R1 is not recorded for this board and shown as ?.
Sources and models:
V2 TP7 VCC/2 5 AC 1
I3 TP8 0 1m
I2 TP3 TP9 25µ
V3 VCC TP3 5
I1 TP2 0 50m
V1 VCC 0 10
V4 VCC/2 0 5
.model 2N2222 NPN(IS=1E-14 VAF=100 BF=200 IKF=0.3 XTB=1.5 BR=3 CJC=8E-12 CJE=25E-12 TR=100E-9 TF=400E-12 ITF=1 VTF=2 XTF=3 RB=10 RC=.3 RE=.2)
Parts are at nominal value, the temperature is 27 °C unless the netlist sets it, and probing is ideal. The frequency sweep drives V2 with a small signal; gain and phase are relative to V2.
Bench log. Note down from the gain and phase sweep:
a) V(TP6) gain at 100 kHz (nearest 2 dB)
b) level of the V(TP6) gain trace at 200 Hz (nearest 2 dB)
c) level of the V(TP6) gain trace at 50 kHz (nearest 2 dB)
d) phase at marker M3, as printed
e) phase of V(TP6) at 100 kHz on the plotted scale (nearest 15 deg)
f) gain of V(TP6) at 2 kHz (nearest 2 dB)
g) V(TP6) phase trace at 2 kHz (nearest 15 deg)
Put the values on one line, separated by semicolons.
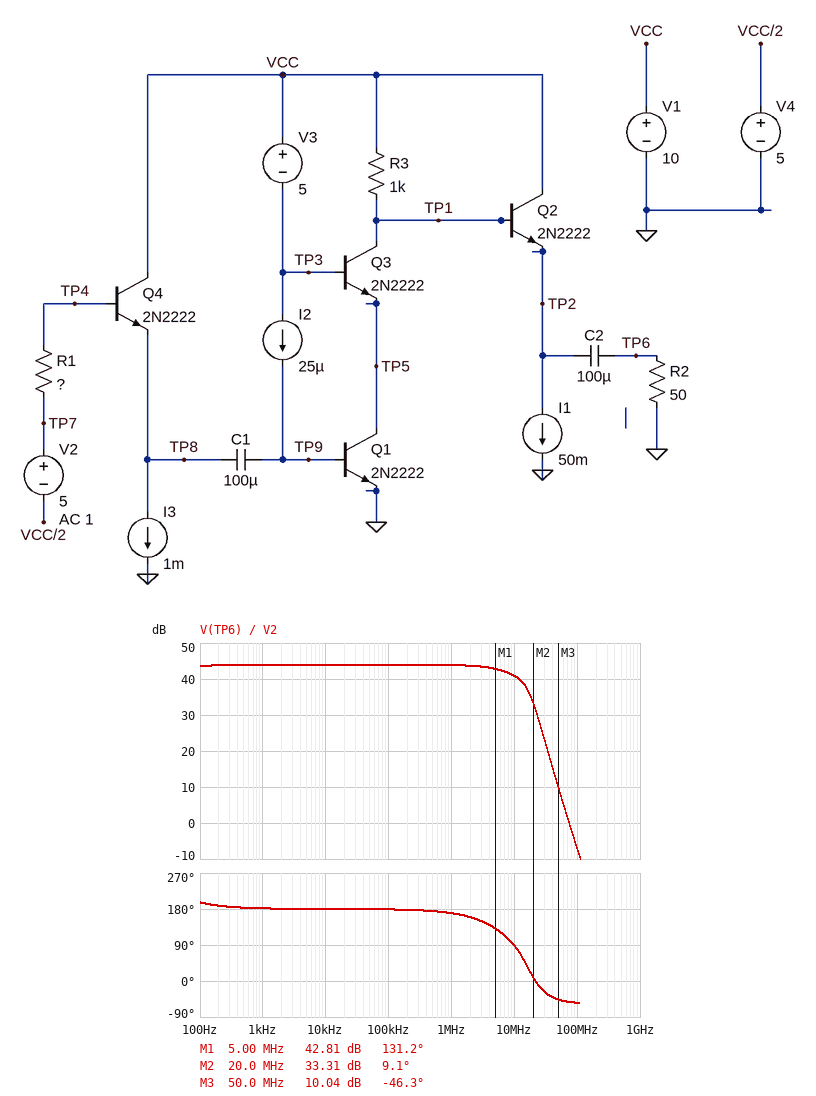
44 dB; 44 dB; 44 dB; -46.3 deg; 180 deg; 44 dB; 180 deg
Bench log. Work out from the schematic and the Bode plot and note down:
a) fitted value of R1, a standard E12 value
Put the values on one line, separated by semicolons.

390 Ω
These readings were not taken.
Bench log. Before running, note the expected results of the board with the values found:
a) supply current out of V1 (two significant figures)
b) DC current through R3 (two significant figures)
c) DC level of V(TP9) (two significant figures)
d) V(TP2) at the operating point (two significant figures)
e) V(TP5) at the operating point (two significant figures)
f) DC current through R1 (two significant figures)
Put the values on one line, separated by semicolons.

56 mA; 5.3 mA; 700 mV; 3.9 V; 4.3 V; 5.0 µA
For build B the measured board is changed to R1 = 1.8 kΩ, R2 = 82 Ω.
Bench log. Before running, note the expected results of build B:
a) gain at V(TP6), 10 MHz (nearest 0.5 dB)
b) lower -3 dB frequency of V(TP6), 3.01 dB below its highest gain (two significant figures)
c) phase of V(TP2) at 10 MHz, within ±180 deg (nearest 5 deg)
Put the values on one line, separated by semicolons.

37.0 dB; 18 Hz; 25 deg
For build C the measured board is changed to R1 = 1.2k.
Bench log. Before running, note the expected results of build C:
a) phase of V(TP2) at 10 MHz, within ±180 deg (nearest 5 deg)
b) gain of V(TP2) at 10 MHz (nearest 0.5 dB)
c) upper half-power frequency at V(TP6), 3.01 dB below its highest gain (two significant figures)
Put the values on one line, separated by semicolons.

40 deg; 39.0 dB; 8.6 MHz
